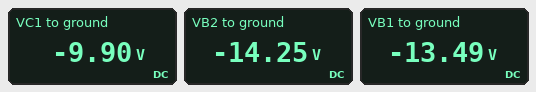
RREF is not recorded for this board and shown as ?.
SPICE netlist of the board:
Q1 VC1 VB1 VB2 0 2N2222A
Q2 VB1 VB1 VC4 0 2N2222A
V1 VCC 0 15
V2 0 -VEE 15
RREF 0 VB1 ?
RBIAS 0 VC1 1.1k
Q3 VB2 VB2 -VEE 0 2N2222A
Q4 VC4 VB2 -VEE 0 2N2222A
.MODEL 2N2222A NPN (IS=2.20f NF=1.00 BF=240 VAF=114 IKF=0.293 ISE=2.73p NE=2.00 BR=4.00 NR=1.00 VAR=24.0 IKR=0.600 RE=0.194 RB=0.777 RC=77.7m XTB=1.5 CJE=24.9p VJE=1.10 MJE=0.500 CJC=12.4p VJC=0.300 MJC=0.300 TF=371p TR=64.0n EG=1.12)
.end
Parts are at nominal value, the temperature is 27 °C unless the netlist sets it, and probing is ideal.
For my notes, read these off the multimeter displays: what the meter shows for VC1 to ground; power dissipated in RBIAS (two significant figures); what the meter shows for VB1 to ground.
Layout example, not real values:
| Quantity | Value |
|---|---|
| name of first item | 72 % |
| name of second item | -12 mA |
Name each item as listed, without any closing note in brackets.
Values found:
| Quantity | Value |
|---|---|
| what the meter shows for VC1 to ground | -9.90 V |
| power dissipated in RBIAS | 89 mW |
| what the meter shows for VB1 to ground | -13.49 V |
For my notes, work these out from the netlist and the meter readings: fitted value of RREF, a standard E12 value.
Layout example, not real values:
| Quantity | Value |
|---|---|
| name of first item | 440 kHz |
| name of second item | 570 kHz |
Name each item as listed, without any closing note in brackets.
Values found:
| Quantity | Value |
|---|---|
| fitted value of RREF, a standard E12 value | 1.5 kΩ |
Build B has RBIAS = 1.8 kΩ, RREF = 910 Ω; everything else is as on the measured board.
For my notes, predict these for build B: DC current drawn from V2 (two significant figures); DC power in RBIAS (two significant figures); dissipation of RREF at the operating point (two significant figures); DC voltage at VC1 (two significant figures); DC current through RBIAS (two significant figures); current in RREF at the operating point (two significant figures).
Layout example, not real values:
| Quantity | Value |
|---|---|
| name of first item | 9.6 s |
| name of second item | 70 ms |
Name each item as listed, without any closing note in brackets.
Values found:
| Quantity | Value |
|---|---|
| DC current drawn from V2 | 23 mA |
| DC power in RBIAS | 110 mW |
| dissipation of RREF at the operating point | 200 mW |
| DC voltage at VC1 | -14 V |
| DC current through RBIAS | 7.9 mA |
| current in RREF at the operating point | 15 mA |
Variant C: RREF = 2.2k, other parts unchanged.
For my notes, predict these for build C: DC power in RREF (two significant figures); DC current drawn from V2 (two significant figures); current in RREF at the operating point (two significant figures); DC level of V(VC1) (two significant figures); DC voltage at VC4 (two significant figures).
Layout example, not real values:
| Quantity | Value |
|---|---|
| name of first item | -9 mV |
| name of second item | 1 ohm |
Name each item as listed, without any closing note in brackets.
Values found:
| Quantity | Value |
|---|---|
| DC power in RREF | 83 mW |
| DC current drawn from V2 | 12 mA |
| current in RREF at the operating point | 6.1 mA |
| DC level of V(VC1) | -6.8 V |
| DC voltage at VC4 | -14 V |
